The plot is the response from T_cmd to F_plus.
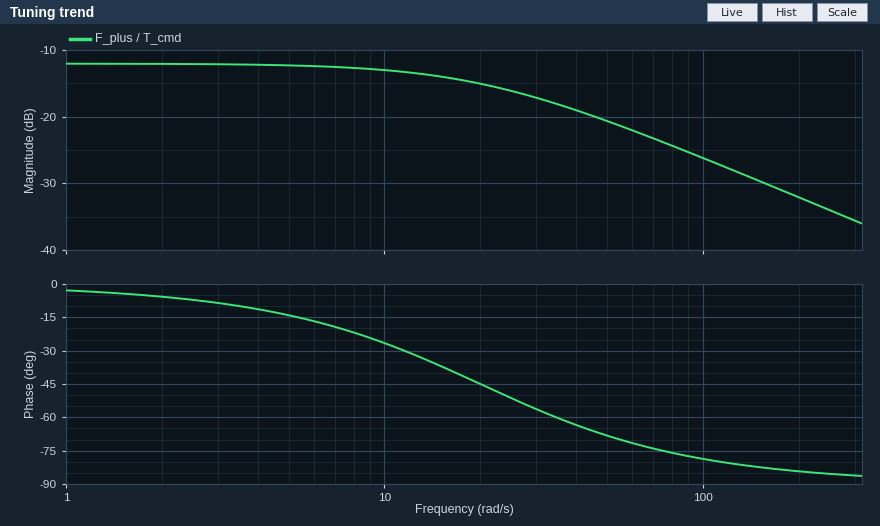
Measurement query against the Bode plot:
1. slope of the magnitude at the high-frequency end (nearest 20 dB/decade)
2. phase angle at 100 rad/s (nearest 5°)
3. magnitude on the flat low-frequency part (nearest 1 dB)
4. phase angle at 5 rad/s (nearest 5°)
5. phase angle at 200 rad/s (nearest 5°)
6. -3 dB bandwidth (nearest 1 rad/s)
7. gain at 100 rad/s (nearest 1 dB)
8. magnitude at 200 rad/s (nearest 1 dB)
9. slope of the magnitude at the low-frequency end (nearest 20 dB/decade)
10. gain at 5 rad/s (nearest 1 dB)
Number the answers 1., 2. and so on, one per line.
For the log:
1. -20 dB/decade
2. -80°
3. -12 dB
4. -15°
5. -85°
6. 20 rad/s
7. -26 dB
8. -32 dB
9. 0 dB/decade
10. -12 dB
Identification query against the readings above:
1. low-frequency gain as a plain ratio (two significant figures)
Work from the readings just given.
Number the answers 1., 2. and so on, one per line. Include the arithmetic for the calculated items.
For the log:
1. 10^(-12 / 20) = 0.25
